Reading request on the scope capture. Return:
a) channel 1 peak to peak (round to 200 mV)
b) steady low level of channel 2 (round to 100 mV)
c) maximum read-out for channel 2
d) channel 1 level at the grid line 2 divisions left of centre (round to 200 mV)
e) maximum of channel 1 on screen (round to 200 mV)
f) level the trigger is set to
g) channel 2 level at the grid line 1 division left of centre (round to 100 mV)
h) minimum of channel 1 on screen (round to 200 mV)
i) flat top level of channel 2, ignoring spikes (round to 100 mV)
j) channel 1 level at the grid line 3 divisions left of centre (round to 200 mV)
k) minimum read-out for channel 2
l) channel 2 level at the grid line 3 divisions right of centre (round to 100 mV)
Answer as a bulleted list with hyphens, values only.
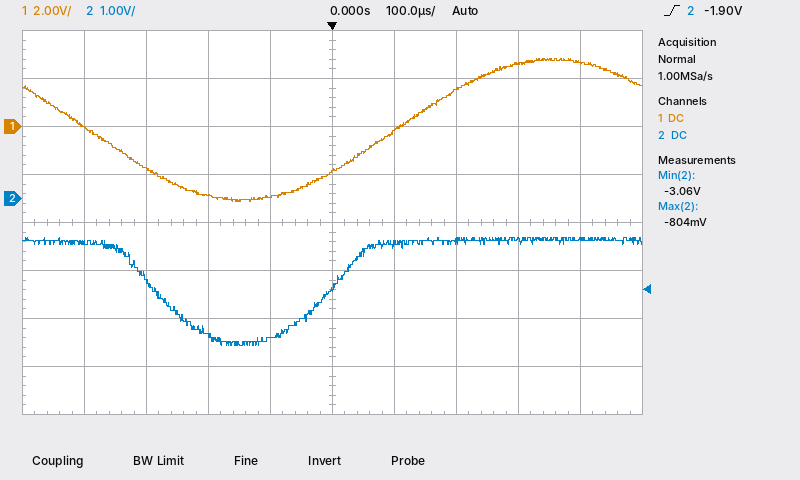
- 6.0 V
- -3.0 V
- -804 mV
- -2.8 V
- 2.8 V
- -1.90 V
- -2.9 V
- -3.2 V
- -900 mV
- -1.8 V
- -3.06 V
- -900 mV
